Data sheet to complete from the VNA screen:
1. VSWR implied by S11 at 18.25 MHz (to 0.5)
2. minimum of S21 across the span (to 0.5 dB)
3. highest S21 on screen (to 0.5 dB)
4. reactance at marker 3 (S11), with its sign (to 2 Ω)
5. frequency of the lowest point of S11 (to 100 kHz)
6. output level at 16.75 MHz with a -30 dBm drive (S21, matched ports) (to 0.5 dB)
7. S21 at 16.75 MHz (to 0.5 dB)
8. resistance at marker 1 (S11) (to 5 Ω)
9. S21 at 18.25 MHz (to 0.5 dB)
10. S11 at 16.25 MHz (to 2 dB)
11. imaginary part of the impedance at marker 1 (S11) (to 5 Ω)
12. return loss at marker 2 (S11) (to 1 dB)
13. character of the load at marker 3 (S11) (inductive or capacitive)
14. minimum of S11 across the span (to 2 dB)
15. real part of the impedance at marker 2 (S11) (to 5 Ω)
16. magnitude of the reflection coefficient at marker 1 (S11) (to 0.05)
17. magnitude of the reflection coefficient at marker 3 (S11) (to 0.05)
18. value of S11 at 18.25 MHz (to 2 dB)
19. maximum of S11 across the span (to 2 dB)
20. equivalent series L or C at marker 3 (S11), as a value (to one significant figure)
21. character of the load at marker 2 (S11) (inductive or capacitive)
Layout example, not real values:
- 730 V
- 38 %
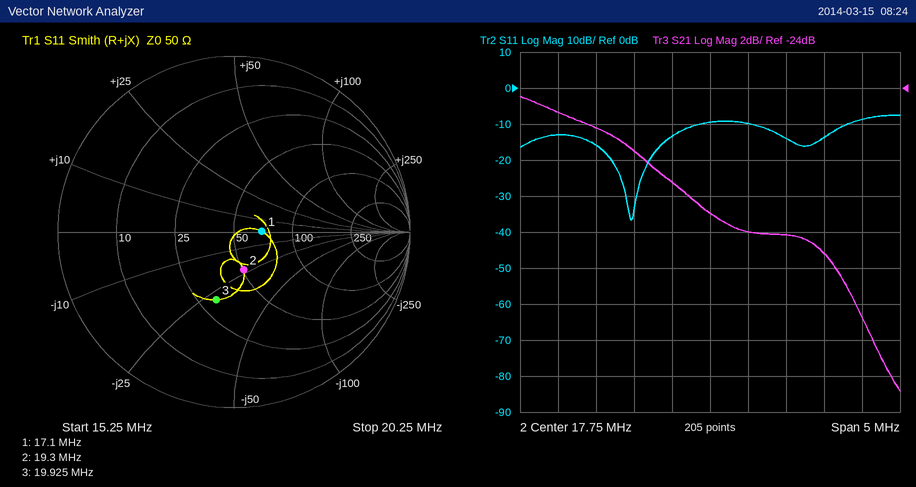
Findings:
- 2.0
- -41.0 dB
- -24.5 dB
- -28 Ω
- 16.7 MHz
- -57.5 dBm
- -27.5 dB
- 70 Ω
- -32.0 dB
- -16 dB
- 0 Ω
- 13 dB
- capacitive
- -36 dB
- 50 Ω
- 0.15
- 0.40
- -10 dB
- -8 dB
- 300 pF
- capacitive
